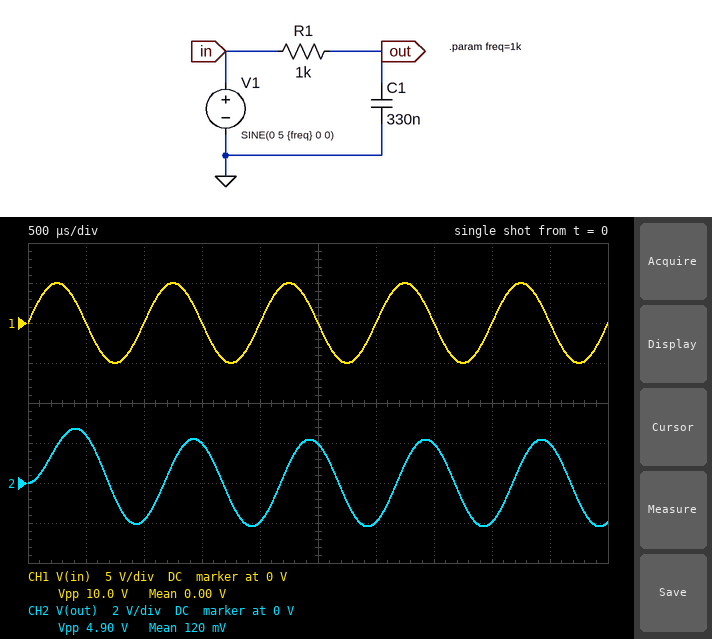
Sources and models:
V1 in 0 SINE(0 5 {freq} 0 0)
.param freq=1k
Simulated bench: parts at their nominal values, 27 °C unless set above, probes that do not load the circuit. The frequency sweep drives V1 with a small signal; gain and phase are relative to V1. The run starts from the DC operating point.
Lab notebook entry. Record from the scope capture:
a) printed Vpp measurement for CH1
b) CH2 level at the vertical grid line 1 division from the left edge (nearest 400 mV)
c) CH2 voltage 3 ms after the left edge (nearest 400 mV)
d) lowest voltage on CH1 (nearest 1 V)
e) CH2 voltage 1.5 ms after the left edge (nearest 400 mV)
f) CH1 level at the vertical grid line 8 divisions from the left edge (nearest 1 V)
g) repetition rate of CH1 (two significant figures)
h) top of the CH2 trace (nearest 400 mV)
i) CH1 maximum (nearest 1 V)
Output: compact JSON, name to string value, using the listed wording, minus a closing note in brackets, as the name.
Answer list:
{"printed Vpp measurement for CH1": "10.0 V", "CH2 level at the vertical grid line 1 division from the left edge": "2.4 V", "CH2 voltage 3 ms after the left edge": "-2.0 V", "lowest voltage on CH1": "-5 V", "CH2 voltage 1.5 ms after the left edge": "2.0 V", "CH1 level at the vertical grid line 8 divisions from the left edge": "0 V", "repetition rate of CH1": "1.0 kHz", "top of the CH2 trace": "2.8 V", "CH1 maximum": "5 V"}
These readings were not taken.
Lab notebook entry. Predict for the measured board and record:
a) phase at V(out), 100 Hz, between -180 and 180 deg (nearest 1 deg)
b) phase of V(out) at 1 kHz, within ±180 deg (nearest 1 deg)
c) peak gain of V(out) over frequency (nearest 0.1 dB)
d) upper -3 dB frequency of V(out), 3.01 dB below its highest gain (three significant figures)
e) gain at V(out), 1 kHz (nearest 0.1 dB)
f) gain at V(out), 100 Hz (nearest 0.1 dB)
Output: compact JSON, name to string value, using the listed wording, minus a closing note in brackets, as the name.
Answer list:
{"phase at V(out), 100 Hz, between -180 and 180 deg": "-12 deg", "phase of V(out) at 1 kHz, within ±180 deg": "-64 deg", "peak gain of V(out) over frequency": "0 dB", "upper -3 dB frequency of V(out), 3.01 dB below its highest gain": "482 Hz", "gain at V(out), 1 kHz": "-7.2 dB", "gain at V(out), 100 Hz": "-0.2 dB"}
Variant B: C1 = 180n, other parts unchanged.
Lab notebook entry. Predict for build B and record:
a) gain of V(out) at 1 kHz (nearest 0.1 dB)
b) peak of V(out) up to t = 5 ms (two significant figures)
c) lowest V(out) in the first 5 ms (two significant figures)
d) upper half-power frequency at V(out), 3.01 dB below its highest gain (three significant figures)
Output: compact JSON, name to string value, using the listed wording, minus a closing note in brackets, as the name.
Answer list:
{"gain of V(out) at 1 kHz": "-3.6 dB", "peak of V(out) up to t = 5 ms": "3.6 V", "lowest V(out) in the first 5 ms": "-3.3 V", "upper half-power frequency at V(out), 3.01 dB below its highest gain": "884 Hz"}
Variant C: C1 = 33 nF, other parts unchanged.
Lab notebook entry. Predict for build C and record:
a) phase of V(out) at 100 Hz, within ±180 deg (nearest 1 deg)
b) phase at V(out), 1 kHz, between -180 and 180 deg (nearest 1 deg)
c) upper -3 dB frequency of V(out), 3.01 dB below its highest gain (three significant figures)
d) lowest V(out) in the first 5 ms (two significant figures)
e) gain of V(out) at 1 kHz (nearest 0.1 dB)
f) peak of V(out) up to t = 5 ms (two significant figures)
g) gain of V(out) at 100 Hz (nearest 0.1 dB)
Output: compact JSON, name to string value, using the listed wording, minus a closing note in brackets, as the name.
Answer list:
{"phase of V(out) at 100 Hz, within ±180 deg": "-1 deg", "phase at V(out), 1 kHz, between -180 and 180 deg": "-12 deg", "upper -3 dB frequency of V(out), 3.01 dB below its highest gain": "4.82 kHz", "lowest V(out) in the first 5 ms": "-4.9 V", "gain of V(out) at 1 kHz": "-0.2 dB", "peak of V(out) up to t = 5 ms": "4.9 V", "gain of V(out) at 100 Hz": "0 dB"}
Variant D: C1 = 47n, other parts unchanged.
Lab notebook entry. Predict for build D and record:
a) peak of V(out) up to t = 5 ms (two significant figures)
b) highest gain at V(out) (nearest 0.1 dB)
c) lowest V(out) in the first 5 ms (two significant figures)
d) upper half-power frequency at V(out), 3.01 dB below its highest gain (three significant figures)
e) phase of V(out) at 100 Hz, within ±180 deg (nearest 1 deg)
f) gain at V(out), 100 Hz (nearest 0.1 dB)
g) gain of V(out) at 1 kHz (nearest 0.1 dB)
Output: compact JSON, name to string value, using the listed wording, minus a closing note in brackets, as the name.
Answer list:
{"peak of V(out) up to t = 5 ms": "4.8 V", "highest gain at V(out)": "0 dB", "lowest V(out) in the first 5 ms": "-4.8 V", "upper half-power frequency at V(out), 3.01 dB below its highest gain": "3.39 kHz", "phase of V(out) at 100 Hz, within ±180 deg": "-2 deg", "gain at V(out), 100 Hz": "0 dB", "gain of V(out) at 1 kHz": "-0.4 dB"}
